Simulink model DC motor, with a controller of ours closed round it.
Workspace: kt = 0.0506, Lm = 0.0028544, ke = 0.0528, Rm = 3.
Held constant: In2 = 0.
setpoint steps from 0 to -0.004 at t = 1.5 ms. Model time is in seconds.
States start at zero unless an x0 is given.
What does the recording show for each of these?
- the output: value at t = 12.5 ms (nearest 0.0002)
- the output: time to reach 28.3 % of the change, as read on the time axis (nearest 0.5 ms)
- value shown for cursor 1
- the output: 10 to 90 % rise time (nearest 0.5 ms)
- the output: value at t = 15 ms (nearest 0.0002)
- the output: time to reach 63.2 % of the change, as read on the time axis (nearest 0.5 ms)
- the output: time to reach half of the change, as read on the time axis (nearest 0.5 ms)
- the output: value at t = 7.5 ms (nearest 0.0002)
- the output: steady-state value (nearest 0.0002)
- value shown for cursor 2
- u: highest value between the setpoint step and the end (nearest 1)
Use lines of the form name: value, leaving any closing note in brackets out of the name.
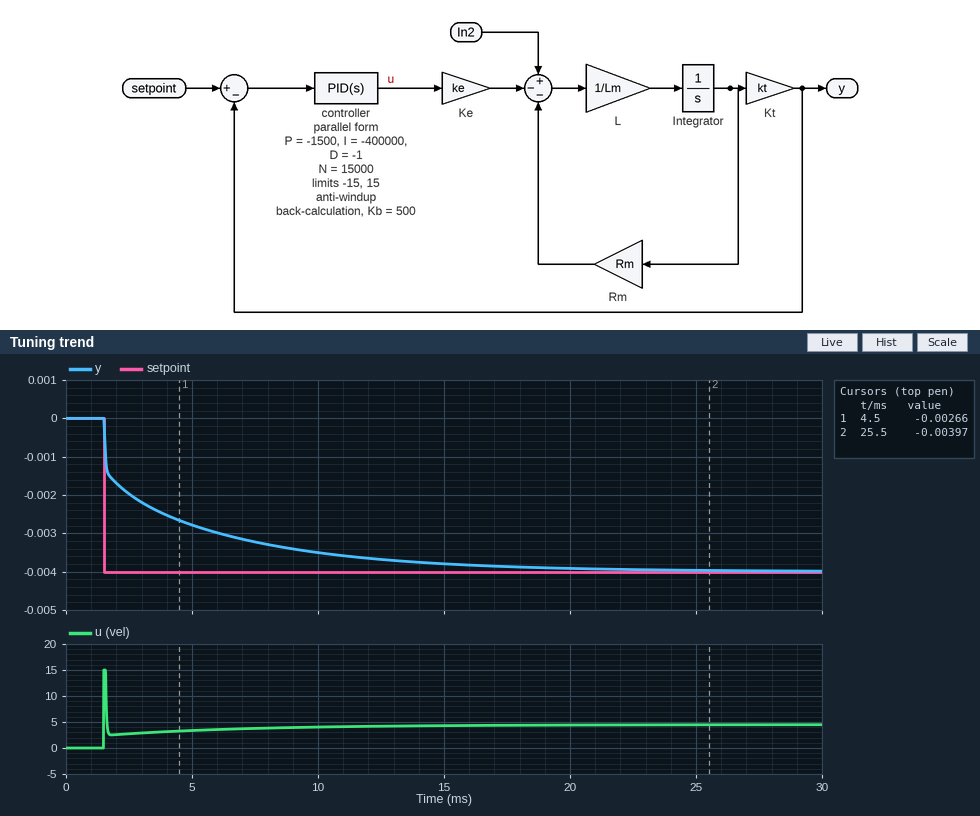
the output: value at t = 12.5 ms: -0.0036
the output: time to reach 28.3 % of the change, as read on the time axis: 1.5 ms
value shown for cursor 1: -0.00266
the output: 10 to 90 % rise time: 9.5 ms
the output: value at t = 15 ms: -0.0038
the output: time to reach 63.2 % of the change, as read on the time axis: 4.0 ms
the output: time to reach half of the change, as read on the time axis: 2.5 ms
the output: value at t = 7.5 ms: -0.0032
the output: steady-state value: -0.0040
value shown for cursor 2: -0.00397
u: highest value between the setpoint step and the end: 15
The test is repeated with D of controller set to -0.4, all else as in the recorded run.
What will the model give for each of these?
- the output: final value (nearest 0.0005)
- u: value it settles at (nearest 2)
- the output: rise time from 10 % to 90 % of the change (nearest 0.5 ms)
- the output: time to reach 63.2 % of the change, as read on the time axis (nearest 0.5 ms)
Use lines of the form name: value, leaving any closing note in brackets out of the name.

the output: final value: -0.0040
u: value it settles at: 4
the output: rise time from 10 % to 90 % of the change: 9.0 ms
the output: time to reach 63.2 % of the change, as read on the time axis: 3.0 ms
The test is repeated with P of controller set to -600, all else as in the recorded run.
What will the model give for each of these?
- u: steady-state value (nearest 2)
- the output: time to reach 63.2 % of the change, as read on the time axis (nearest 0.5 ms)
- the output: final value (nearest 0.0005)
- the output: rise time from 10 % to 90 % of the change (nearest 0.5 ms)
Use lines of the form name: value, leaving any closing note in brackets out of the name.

u: steady-state value: 4
the output: time to reach 63.2 % of the change, as read on the time axis: 5.5 ms
the output: final value: -0.0040
the output: rise time from 10 % to 90 % of the change: 7.5 ms
